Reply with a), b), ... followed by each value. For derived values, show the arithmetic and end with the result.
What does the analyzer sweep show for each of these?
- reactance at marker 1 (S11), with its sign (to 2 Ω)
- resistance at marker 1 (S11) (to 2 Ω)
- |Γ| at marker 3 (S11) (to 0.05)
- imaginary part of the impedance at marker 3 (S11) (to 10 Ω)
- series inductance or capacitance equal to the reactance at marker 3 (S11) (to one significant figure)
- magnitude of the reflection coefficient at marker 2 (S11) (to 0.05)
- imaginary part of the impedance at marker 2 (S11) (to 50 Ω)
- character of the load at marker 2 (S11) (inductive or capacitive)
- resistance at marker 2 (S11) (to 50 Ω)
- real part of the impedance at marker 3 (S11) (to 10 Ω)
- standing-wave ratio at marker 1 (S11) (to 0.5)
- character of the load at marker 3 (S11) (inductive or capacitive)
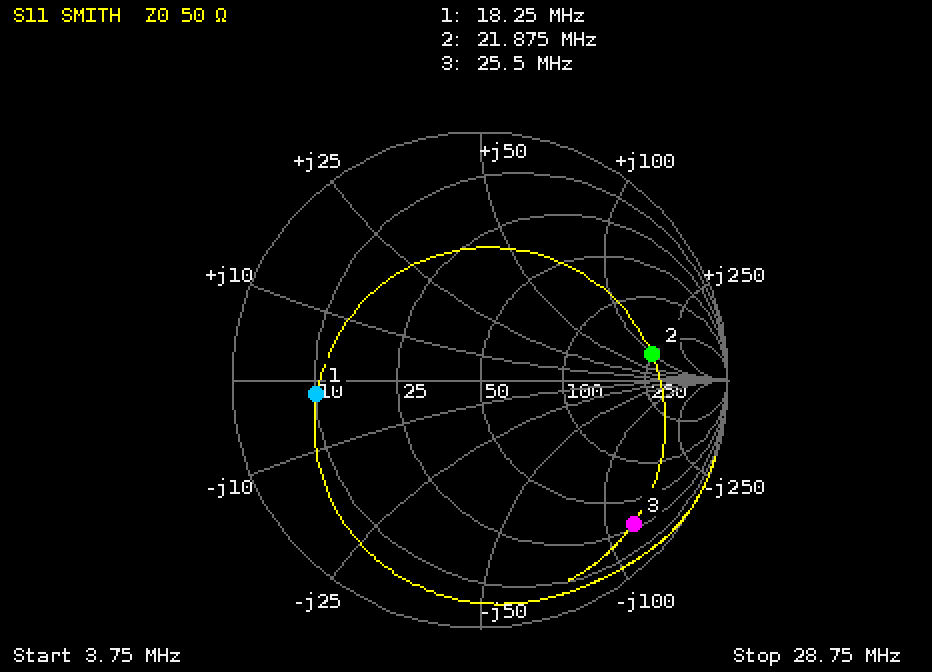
a) -2 Ω
b) 10 Ω
c) 0.85
d) -120 Ω
e) C = 1/(2π × 25.5 MHz × 120 Ω) ≈ 52.0 pF, so 50 pF to one significant figure
f) 0.70
g) +100 Ω
h) inductive
i) 250 Ω
j) 30 Ω
k) 5.0
l) capacitive
